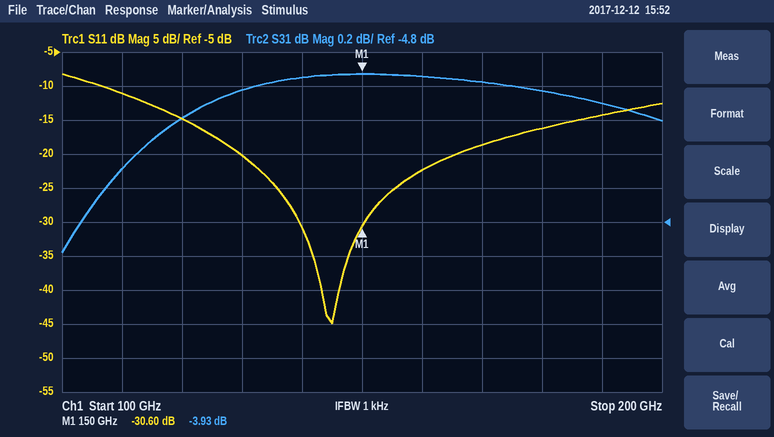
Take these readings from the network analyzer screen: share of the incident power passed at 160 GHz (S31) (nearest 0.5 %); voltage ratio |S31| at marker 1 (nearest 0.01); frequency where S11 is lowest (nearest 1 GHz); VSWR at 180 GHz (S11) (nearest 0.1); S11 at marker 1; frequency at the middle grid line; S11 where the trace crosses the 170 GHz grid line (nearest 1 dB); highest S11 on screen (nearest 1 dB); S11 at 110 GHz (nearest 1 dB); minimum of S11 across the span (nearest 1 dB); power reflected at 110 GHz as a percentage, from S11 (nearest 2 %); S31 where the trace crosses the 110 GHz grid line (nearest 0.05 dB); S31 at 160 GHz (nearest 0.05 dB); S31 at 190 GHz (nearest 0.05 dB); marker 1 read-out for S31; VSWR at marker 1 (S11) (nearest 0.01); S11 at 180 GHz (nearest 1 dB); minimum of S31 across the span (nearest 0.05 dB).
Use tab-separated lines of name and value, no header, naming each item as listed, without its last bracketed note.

share of the incident power passed at 160 GHz (S31)	40.5 %
voltage ratio |S31| at marker 1	0.64
frequency where S11 is lowest	145 GHz
VSWR at 180 GHz (S11)	1.4
S11 at marker 1	-30.60 dB
frequency at the middle grid line	150 GHz
S11 where the trace crosses the 170 GHz grid line	-19 dB
highest S11 on screen	-8 dB
S11 at 110 GHz	-11 dB
minimum of S11 across the span	-45 dB
power reflected at 110 GHz as a percentage, from S11	8 %
S31 where the trace crosses the 110 GHz grid line	-4.50 dB
S31 at 160 GHz	-3.95 dB
S31 at 190 GHz	-4.10 dB
marker 1 read-out for S31	-3.93 dB
VSWR at marker 1 (S11)	1.06
S11 at 180 GHz	-16 dB
minimum of S31 across the span	-5.00 dB
